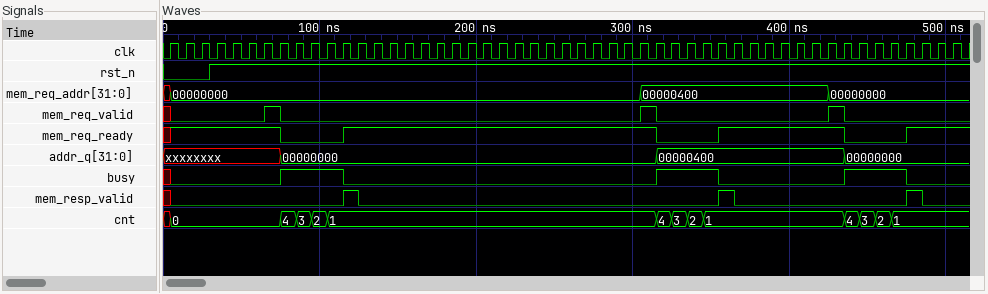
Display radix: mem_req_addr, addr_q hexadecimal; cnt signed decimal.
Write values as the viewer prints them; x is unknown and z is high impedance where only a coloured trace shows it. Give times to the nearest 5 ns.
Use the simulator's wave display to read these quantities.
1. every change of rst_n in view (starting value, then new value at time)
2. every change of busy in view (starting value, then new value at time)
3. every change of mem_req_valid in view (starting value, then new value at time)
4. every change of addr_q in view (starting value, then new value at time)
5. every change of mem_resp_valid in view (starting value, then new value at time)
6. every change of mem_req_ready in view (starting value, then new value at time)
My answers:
0, 1 at 30 ns
x, 0 at 5 ns, 1 at 75 ns, 0 at 115 ns, 1 at 315 ns, 0 at 355 ns, 1 at 435 ns, 0 at 475 ns
x, 0 at 5 ns, 1 at 65 ns, 0 at 75 ns, 1 at 305 ns, 0 at 315 ns, 1 at 425 ns, 0 at 435 ns
xxxxxxxx, 00000000 at 75 ns, 00000400 at 315 ns, 00000000 at 435 ns
x, 0 at 5 ns, 1 at 115 ns, 0 at 125 ns, 1 at 355 ns, 0 at 365 ns, 1 at 475 ns, 0 at 485 ns
x, 1 at 5 ns, 0 at 75 ns, 1 at 115 ns, 0 at 315 ns, 1 at 355 ns, 0 at 435 ns, 1 at 475 ns
